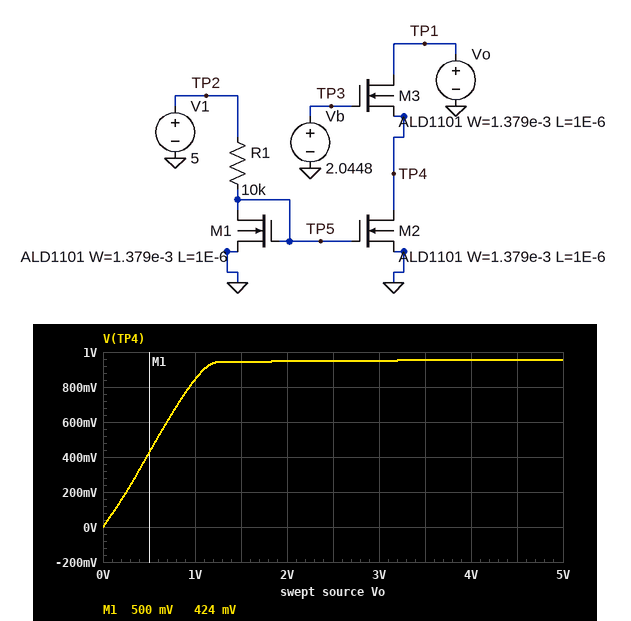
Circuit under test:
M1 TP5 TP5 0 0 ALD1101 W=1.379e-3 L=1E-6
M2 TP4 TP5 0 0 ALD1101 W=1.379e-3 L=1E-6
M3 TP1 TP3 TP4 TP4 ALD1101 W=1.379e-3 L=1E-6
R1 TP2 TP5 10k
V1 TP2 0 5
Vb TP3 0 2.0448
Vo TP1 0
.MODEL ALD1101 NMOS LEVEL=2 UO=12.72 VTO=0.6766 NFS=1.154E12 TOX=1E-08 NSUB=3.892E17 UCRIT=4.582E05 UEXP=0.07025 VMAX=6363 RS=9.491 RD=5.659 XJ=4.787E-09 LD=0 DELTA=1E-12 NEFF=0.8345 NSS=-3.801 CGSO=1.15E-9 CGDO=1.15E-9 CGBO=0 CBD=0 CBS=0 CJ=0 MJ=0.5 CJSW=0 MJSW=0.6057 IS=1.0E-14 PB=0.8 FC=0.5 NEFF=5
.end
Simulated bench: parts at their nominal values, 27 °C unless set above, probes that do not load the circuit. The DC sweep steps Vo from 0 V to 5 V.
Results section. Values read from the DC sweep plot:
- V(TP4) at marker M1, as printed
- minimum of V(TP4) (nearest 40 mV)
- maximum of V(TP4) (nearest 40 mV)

424 mV
0 V
960 mV
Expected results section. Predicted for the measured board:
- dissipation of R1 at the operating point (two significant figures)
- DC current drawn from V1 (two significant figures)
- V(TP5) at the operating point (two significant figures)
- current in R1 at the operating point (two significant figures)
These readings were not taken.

1.5 mW
390 µA
1.1 V
390 µA
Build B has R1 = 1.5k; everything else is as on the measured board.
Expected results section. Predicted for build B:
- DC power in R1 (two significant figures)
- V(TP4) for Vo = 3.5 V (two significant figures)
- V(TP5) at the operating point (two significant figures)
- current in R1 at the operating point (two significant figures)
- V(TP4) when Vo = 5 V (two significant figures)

7.2 mW
440 mV
1.7 V
2.2 mA
450 mV
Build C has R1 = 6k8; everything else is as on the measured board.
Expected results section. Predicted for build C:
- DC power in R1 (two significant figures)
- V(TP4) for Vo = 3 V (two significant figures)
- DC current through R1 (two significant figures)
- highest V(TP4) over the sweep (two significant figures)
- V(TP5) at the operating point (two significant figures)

2.1 mW
860 mV
560 µA
870 mV
1.2 V
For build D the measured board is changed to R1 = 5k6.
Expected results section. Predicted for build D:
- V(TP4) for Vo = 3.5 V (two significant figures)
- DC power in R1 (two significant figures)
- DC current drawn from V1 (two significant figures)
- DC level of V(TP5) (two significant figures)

820 mV
2.5 mW
670 µA
1.2 V
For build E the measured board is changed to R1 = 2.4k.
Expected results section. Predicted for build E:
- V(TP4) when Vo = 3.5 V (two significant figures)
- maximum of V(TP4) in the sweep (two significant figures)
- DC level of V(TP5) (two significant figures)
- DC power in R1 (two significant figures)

550 mV
560 mV
1.5 V
5.1 mW
